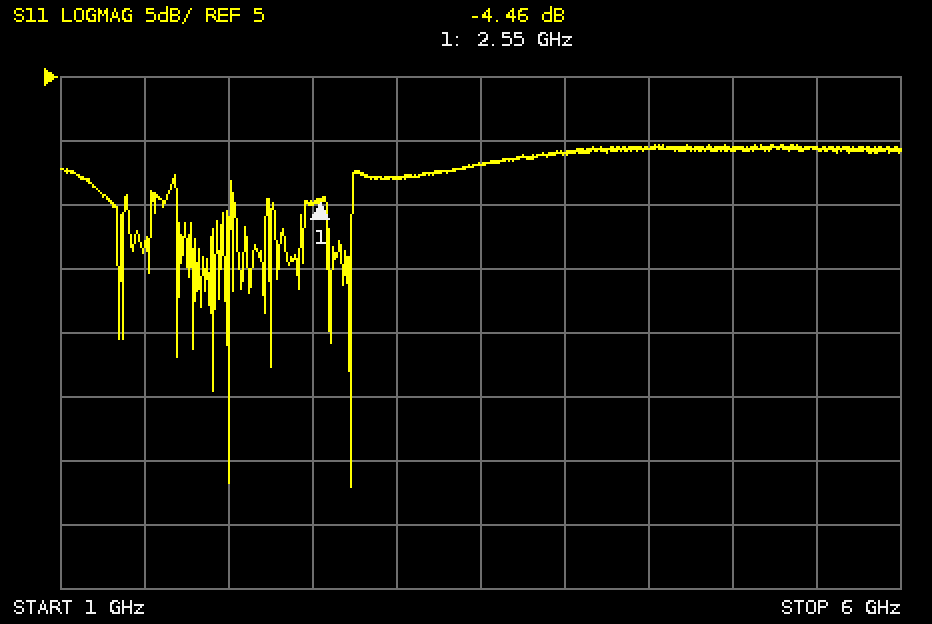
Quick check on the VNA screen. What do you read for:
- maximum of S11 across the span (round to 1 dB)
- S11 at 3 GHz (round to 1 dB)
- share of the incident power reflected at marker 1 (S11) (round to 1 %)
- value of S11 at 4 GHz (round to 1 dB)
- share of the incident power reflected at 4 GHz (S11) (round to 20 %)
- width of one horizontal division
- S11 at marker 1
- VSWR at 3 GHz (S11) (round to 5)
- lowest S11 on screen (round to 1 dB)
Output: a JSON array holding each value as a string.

["0 dB", "-3 dB", "36 %", "-1 dB", "80 %", "500 MHz", "-4.46 dB", "5", "-27 dB"]
